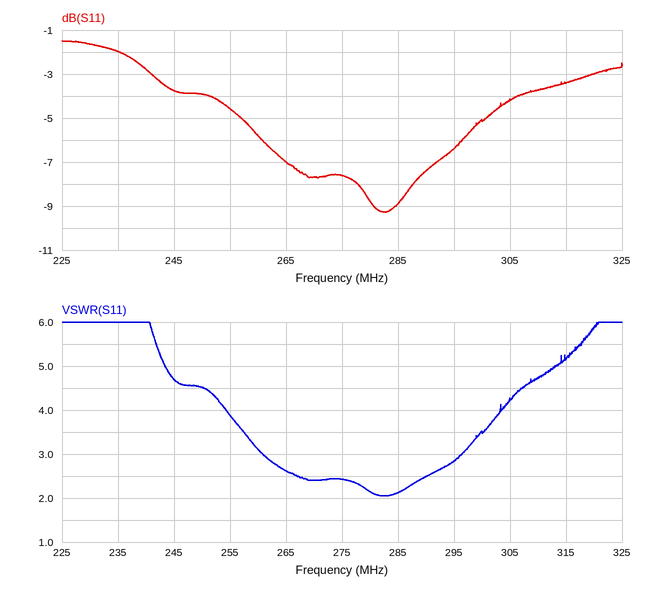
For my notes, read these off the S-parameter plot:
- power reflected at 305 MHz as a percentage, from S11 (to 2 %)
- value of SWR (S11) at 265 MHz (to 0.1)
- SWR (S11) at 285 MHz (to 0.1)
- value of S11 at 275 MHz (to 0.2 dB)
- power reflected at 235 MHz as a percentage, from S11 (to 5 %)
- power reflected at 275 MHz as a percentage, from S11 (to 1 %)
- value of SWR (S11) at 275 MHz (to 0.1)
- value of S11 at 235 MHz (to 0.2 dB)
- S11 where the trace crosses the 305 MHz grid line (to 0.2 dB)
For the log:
38 %
2.6
2.1
-7.6 dB
65 %
17 %
2.4
-2.0 dB
-4.2 dB
